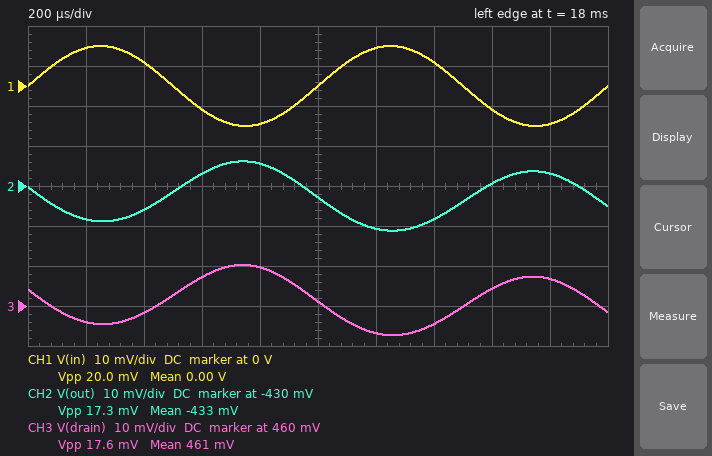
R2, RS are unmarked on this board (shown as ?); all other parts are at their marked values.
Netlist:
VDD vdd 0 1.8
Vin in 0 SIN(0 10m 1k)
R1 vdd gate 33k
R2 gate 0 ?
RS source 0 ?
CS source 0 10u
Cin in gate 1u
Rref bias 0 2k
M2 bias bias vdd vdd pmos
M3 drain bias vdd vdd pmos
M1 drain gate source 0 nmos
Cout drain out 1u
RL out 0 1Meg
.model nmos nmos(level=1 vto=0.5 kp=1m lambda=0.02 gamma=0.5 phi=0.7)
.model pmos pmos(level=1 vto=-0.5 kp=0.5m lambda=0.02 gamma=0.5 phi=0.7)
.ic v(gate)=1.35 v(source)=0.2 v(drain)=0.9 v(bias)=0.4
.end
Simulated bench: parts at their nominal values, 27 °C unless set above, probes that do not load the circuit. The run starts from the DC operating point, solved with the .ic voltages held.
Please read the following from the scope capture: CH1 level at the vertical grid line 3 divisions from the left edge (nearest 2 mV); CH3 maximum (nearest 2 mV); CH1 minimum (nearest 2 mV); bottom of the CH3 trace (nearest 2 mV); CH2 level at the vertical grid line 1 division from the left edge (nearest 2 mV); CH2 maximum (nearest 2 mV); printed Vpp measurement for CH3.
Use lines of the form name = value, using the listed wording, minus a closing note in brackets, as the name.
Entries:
CH1 level at the vertical grid line 3 divisions from the left edge = -6 mV
CH3 maximum = 470 mV
CH1 minimum = -10 mV
bottom of the CH3 trace = 452 mV
CH2 level at the vertical grid line 1 division from the left edge = -438 mV
CH2 maximum = -424 mV
printed Vpp measurement for CH3 = 17.6 mV
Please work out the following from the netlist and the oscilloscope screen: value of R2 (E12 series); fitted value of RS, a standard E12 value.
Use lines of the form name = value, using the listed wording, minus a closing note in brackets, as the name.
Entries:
value of R2 = 150 kΩ
fitted value of RS, a standard E12 value = 560 Ω
